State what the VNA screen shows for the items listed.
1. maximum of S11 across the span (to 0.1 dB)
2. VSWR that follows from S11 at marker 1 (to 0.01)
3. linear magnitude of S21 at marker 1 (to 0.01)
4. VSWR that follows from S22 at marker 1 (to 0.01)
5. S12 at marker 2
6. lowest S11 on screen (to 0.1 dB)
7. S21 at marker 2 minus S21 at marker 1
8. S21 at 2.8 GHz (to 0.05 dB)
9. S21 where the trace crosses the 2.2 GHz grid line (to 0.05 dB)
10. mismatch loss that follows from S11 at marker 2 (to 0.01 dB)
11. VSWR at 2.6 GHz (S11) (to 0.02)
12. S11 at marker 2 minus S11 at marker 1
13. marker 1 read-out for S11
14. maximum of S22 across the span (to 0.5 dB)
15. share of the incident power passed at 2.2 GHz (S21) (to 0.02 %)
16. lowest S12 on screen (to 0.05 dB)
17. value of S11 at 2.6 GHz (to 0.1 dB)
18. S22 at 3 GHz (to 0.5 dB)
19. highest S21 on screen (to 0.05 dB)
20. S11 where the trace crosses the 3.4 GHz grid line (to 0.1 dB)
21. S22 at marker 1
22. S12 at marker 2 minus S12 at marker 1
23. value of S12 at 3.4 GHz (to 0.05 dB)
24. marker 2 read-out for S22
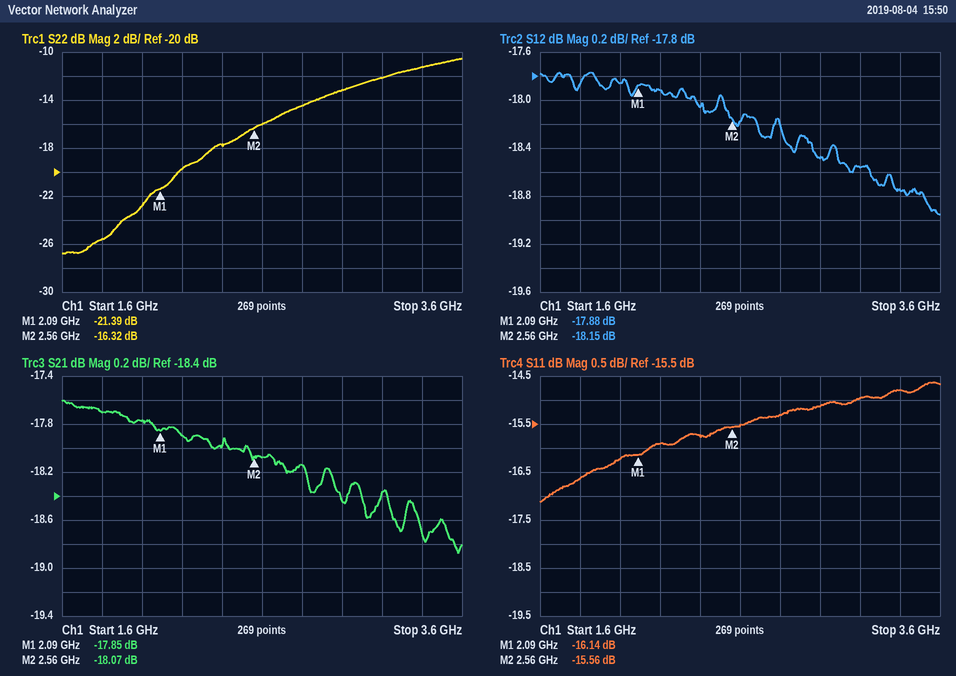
-14.6 dB
1.37
0.13
1.19
-18.15 dB
-17.1 dB
-0.22 dB
-18.15 dB
-17.90 dB
0.12 dB
1.40
0.58 dB
-16.14 dB
-10.5 dB
1.62 %
-18.95 dB
-15.5 dB
-13.0 dB
-17.60 dB
-14.8 dB
-21.39 dB
-0.27 dB
-18.75 dB
-16.32 dB
